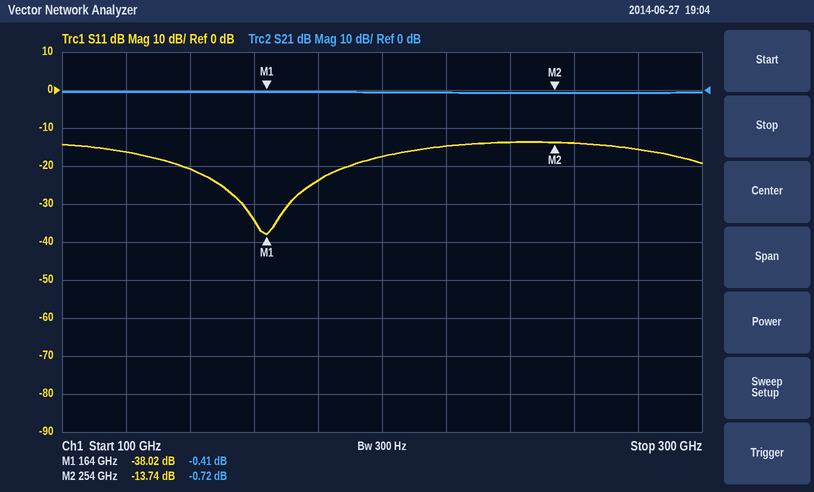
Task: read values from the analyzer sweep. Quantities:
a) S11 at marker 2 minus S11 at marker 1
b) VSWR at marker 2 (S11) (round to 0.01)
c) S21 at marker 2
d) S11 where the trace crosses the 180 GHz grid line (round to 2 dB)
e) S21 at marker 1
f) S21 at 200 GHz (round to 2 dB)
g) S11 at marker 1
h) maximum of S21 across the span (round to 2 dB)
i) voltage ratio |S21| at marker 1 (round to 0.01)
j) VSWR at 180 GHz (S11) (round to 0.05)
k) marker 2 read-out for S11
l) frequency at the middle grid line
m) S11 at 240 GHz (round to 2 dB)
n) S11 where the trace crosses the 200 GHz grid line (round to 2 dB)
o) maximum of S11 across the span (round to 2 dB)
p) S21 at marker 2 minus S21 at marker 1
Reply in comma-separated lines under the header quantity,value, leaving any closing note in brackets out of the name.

quantity,value
S11 at marker 2 minus S11 at marker 1,24.28 dB
VSWR at marker 2 (S11),1.52
S21 at marker 2,-0.72 dB
S11 where the trace crosses the 180 GHz grid line,-24 dB
S21 at marker 1,-0.41 dB
S21 at 200 GHz,0 dB
S11 at marker 1,-38.02 dB
maximum of S21 across the span,0 dB
voltage ratio |S21| at marker 1,0.95
VSWR at 180 GHz (S11),1.15
marker 2 read-out for S11,-13.74 dB
frequency at the middle grid line,200 GHz
S11 at 240 GHz,-14 dB
S11 where the trace crosses the 200 GHz grid line,-18 dB
maximum of S11 across the span,-14 dB
S21 at marker 2 minus S21 at marker 1,-0.31 dB
